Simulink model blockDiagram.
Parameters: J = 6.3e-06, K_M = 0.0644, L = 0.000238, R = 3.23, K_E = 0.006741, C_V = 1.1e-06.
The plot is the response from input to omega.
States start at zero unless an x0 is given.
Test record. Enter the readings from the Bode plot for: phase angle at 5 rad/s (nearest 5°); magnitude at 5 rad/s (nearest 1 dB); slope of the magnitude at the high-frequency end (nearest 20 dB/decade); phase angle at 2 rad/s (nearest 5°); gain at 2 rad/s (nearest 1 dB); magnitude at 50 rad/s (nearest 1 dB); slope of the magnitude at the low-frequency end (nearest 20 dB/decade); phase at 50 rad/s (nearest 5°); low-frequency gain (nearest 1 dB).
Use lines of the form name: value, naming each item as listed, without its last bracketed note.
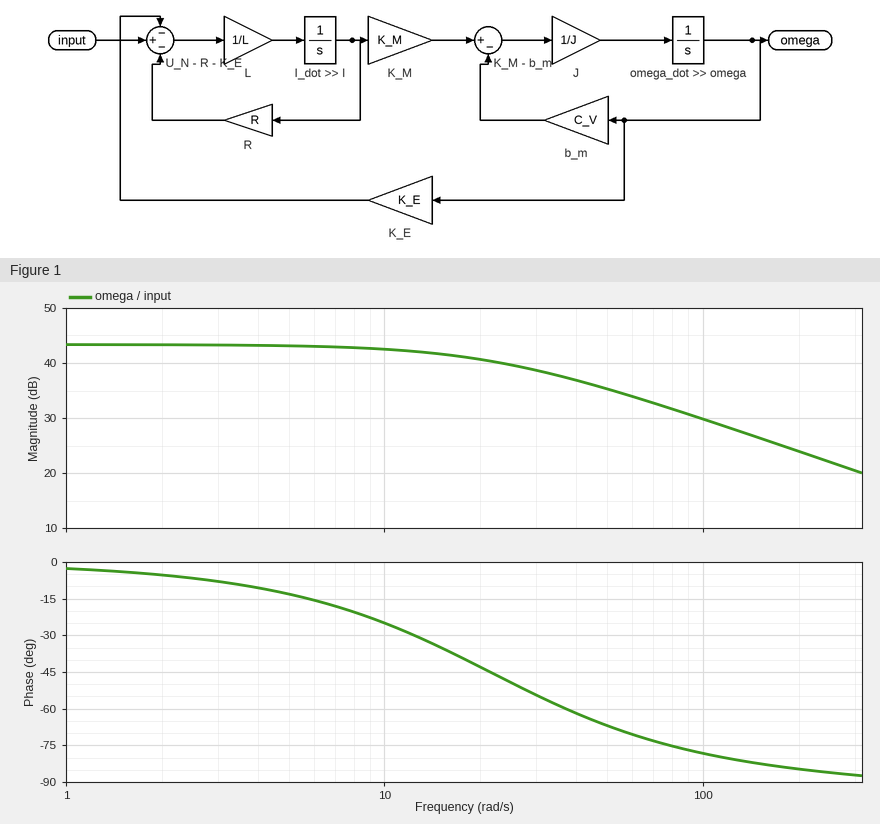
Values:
phase angle at 5 rad/s: -15°
magnitude at 5 rad/s: 43 dB
slope of the magnitude at the high-frequency end: -20 dB/decade
phase angle at 2 rad/s: -5°
gain at 2 rad/s: 43 dB
magnitude at 50 rad/s: 35 dB
slope of the magnitude at the low-frequency end: 0 dB/decade
phase at 50 rad/s: -65°
low-frequency gain: 43 dB
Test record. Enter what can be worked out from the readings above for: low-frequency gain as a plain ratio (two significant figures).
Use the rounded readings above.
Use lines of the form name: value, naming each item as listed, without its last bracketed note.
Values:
low-frequency gain as a plain ratio: 140
